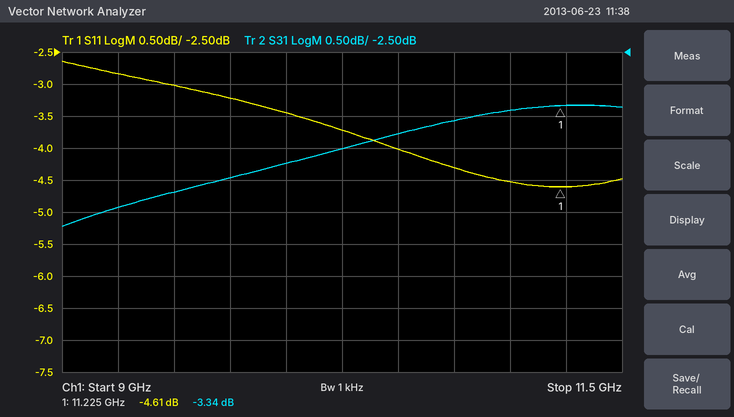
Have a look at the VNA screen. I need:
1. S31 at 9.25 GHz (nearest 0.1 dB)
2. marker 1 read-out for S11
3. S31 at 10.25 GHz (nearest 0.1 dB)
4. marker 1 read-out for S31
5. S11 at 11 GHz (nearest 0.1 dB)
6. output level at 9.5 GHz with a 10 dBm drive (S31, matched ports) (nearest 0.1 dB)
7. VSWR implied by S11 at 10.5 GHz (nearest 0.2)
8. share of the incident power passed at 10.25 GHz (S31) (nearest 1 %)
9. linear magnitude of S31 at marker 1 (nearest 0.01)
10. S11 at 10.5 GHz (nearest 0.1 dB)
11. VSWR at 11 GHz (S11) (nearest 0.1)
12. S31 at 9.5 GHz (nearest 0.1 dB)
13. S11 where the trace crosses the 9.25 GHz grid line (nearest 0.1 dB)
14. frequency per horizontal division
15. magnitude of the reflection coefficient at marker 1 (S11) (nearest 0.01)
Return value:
-4.9 dB
-4.61 dB
-4.0 dB
-3.34 dB
-4.5 dB
5.3 dBm
4.4
40 %
0.68
-4.0 dB
3.9
-4.7 dB
-2.8 dB
250 MHz
0.59
